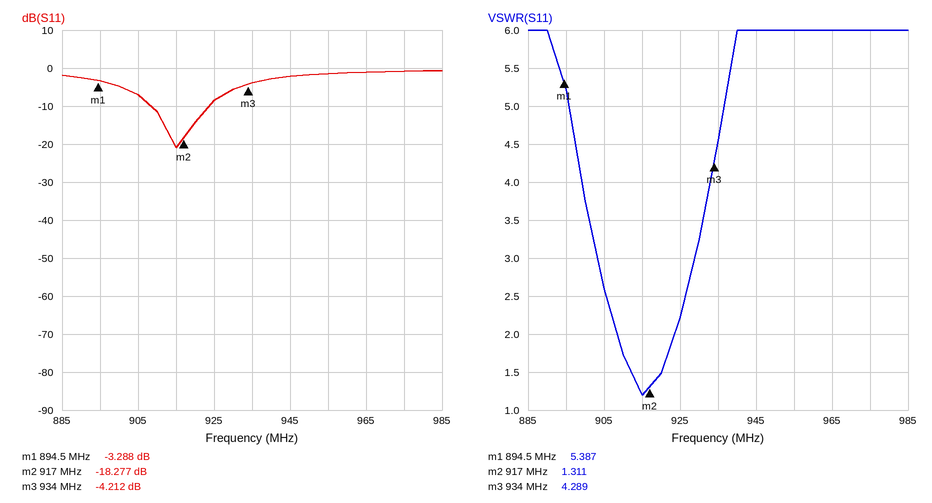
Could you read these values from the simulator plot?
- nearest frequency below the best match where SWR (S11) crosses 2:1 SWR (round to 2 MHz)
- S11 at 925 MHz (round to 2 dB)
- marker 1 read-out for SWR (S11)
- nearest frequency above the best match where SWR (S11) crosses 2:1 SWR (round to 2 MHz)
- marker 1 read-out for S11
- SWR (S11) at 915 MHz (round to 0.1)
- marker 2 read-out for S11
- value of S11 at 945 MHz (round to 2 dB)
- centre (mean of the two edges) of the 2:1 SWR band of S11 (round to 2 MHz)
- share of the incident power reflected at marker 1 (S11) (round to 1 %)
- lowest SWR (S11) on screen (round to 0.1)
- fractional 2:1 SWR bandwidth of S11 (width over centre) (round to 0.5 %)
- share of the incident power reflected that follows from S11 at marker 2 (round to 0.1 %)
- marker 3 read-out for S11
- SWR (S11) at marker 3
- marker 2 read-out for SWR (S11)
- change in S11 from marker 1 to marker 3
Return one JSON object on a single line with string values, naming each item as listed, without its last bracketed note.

{"nearest frequency below the best match where SWR (S11) crosses 2:1 SWR": "908 MHz", "S11 at 925 MHz": "-8 dB", "marker 1 read-out for SWR": "5.387", "nearest frequency above the best match where SWR (S11) crosses 2:1 SWR": "924 MHz", "marker 1 read-out for S11": "-3.288 dB", "SWR (S11) at 915 MHz": "1.2", "marker 2 read-out for S11": "-18.277 dB", "value of S11 at 945 MHz": "-2 dB", "centre (mean of the two edges) of the 2:1 SWR band of S11": "916 MHz", "share of the incident power reflected at marker 1 (S11)": "47 %", "lowest SWR (S11) on screen": "1.2", "fractional 2:1 SWR bandwidth of S11 (width over centre)": "1.5 %", "share of the incident power reflected that follows from S11 at marker 2": "1.5 %", "marker 3 read-out for S11": "-4.212 dB", "SWR (S11) at marker 3": "4.289", "marker 2 read-out for SWR": "1.311", "change in S11 from marker 1 to marker 3": "-0.924 dB"}
